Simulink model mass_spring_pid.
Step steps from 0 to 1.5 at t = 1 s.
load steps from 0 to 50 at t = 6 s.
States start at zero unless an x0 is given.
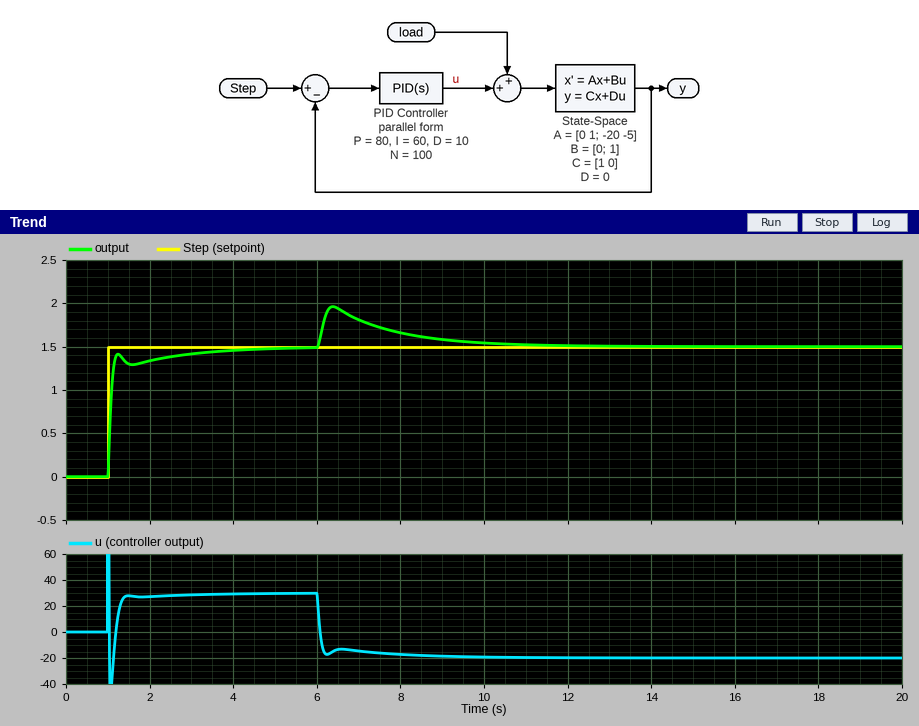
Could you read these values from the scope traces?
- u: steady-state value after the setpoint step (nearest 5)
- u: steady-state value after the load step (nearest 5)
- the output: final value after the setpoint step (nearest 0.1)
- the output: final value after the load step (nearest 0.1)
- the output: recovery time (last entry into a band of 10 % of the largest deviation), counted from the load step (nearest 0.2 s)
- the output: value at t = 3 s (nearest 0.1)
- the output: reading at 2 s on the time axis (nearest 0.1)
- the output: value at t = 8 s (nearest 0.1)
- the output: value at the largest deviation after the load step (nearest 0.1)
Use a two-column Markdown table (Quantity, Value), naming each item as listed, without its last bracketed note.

| Quantity | Value |
|---|---|
| u: steady-state value after the setpoint step | 30 |
| u: steady-state value after the load step | -20 |
| the output: final value after the setpoint step | 1.5 |
| the output: final value after the load step | 1.5 |
| the output: recovery time (last entry into a band of 10 % of the largest deviation), counted from the load step | 3.8 s |
| the output: value at t = 3 s | 1.4 |
| the output: reading at 2 s on the time axis | 1.3 |
| the output: value at t = 8 s | 1.7 |
| the output: value at the largest deviation after the load step | 2.0 |
